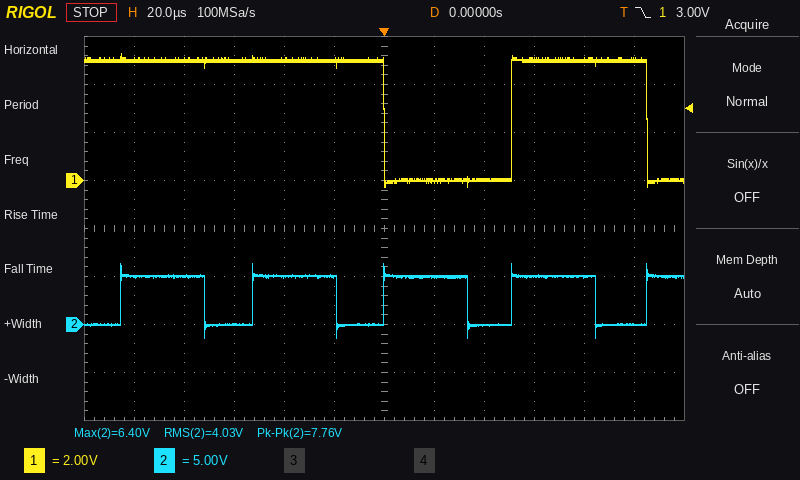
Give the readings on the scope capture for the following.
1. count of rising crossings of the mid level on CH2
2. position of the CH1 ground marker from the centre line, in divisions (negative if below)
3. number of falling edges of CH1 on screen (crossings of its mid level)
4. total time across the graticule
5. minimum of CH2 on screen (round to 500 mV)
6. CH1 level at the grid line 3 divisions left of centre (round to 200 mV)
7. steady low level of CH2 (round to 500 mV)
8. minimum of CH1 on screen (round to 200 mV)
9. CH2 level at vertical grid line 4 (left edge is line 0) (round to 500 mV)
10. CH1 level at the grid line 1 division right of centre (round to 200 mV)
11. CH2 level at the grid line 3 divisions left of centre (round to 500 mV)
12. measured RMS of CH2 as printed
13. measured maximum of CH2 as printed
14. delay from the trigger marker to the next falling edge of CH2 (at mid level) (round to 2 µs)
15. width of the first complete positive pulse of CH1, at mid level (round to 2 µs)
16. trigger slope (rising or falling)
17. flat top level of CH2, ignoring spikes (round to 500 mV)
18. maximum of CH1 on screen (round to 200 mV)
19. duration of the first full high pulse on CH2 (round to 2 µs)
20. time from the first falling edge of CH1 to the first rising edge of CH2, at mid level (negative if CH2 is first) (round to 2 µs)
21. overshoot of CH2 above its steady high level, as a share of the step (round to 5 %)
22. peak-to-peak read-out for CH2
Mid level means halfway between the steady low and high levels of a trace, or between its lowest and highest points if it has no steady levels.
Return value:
5
+1.0 div
2
240 µs
-1.5 V
5.0 V
0.0 V
-200 mV
5.0 V
0.0 V
0.0 V
4.03 V
6.40 V
34 µs
54 µs
falling
5.0 V
5.2 V
34 µs
-106 µs
25 %
7.76 V
